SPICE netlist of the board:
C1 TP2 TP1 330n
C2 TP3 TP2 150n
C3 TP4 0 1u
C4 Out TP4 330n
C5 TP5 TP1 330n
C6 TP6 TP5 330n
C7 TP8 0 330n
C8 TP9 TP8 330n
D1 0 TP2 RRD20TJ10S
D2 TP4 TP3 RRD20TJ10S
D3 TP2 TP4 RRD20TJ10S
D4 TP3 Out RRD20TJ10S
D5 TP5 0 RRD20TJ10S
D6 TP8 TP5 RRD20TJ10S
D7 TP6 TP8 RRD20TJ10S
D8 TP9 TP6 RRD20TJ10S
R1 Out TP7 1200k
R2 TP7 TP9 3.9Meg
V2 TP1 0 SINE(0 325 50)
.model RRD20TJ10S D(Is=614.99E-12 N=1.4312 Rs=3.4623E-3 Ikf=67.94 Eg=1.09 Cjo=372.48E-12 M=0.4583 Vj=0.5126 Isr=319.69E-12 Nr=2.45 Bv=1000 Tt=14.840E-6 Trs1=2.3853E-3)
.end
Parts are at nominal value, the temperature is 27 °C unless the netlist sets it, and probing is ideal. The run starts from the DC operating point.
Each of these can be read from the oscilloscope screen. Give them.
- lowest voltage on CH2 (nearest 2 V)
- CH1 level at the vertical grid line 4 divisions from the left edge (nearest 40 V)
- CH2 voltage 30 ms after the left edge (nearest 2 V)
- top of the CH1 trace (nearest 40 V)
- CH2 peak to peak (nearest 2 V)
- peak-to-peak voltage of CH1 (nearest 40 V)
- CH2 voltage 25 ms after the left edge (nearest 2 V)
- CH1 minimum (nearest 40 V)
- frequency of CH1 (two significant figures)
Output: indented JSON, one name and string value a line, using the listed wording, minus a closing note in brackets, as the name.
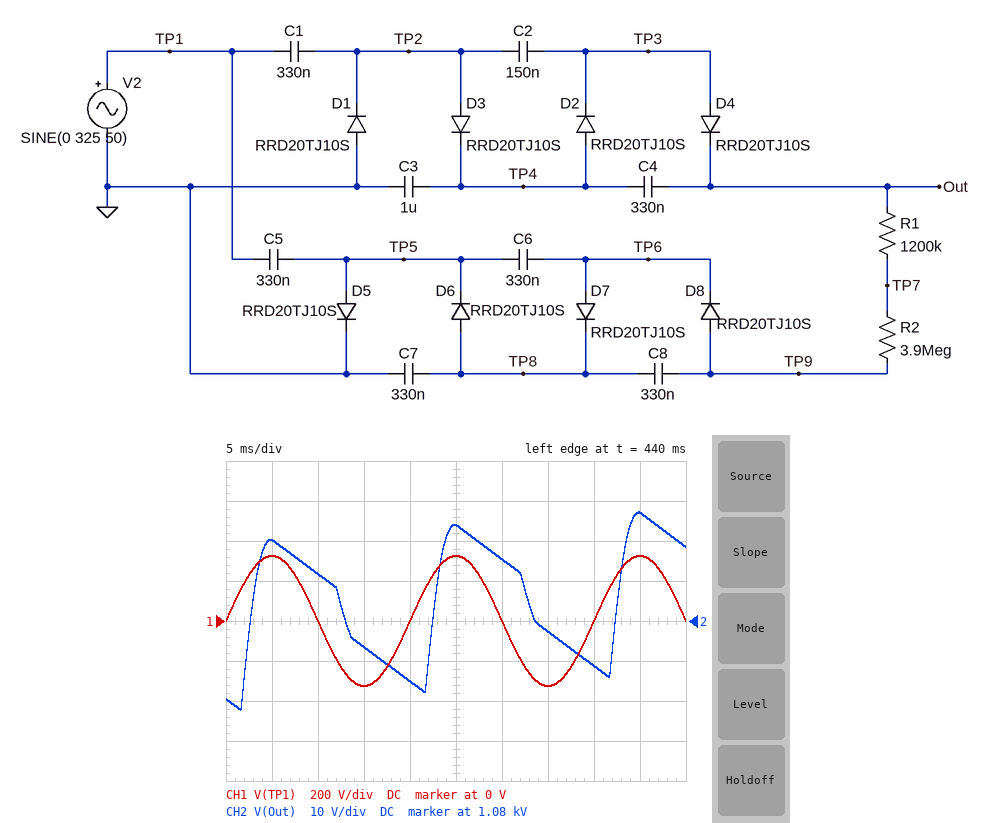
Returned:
{
  "lowest voltage on CH2": "1.058 kV",
  "CH1 level at the vertical grid line 4 divisions from the left edge": "0 V",
  "CH2 voltage 30 ms after the left edge": "1.096 kV",
  "top of the CH1 trace": "320 V",
  "CH2 peak to peak": "50 V",
  "peak-to-peak voltage of CH1": "640 V",
  "CH2 voltage 25 ms after the left edge": "1.104 kV",
  "CH1 minimum": "-320 V",
  "frequency of CH1": "50 Hz"
}
